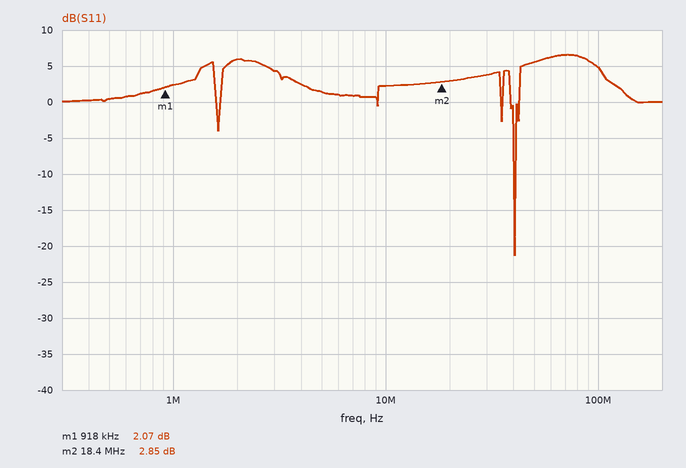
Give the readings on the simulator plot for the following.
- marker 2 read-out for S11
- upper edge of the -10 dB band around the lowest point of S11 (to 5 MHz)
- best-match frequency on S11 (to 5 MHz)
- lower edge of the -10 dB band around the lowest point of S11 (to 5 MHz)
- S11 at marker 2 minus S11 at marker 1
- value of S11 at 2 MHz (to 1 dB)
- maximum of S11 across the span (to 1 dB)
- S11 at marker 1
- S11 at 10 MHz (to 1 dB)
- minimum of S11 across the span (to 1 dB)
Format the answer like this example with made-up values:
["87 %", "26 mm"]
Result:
["2.85 dB", "40 MHz", "40 MHz", "40 MHz", "0.78 dB", "6 dB", "7 dB", "2.07 dB", "2 dB", "-21 dB"]
